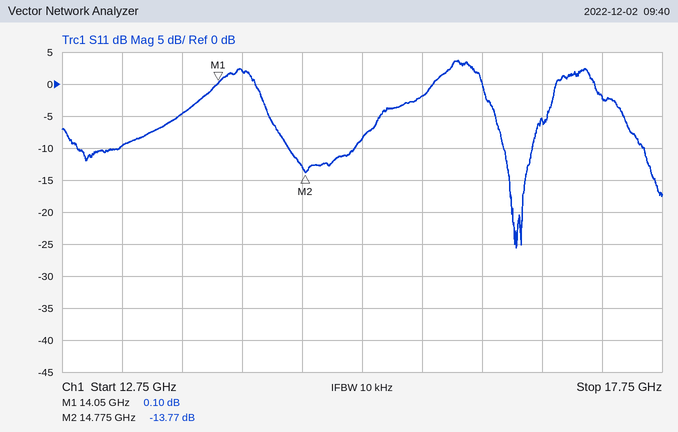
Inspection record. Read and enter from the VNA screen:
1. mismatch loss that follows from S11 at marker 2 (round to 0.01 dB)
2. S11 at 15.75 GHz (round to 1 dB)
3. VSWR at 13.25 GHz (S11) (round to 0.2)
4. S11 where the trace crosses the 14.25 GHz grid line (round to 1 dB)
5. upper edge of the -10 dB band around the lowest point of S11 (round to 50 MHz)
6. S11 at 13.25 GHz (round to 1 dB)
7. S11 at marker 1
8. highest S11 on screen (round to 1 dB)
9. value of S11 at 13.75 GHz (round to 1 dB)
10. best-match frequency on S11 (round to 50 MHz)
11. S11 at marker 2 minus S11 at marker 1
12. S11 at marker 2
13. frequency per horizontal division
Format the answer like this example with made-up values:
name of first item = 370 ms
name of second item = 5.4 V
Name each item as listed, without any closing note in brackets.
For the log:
mismatch loss that follows from S11 at marker 2 = 0.19 dB
S11 at 15.75 GHz = -2 dB
VSWR at 13.25 GHz (S11) = 2.0
S11 where the trace crosses the 14.25 GHz grid line = 2 dB
upper edge of the -10 dB band around the lowest point of S11 = 16.65 GHz
S11 at 13.25 GHz = -10 dB
S11 at marker 1 = 0.10 dB
highest S11 on screen = 4 dB
value of S11 at 13.75 GHz = -5 dB
best-match frequency on S11 = 16.55 GHz
S11 at marker 2 minus S11 at marker 1 = -13.87 dB
S11 at marker 2 = -13.77 dB
frequency per horizontal division = 500 MHz
